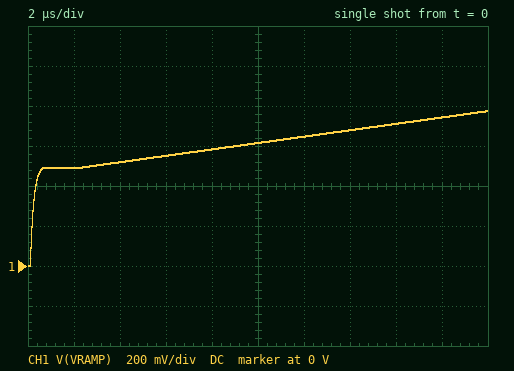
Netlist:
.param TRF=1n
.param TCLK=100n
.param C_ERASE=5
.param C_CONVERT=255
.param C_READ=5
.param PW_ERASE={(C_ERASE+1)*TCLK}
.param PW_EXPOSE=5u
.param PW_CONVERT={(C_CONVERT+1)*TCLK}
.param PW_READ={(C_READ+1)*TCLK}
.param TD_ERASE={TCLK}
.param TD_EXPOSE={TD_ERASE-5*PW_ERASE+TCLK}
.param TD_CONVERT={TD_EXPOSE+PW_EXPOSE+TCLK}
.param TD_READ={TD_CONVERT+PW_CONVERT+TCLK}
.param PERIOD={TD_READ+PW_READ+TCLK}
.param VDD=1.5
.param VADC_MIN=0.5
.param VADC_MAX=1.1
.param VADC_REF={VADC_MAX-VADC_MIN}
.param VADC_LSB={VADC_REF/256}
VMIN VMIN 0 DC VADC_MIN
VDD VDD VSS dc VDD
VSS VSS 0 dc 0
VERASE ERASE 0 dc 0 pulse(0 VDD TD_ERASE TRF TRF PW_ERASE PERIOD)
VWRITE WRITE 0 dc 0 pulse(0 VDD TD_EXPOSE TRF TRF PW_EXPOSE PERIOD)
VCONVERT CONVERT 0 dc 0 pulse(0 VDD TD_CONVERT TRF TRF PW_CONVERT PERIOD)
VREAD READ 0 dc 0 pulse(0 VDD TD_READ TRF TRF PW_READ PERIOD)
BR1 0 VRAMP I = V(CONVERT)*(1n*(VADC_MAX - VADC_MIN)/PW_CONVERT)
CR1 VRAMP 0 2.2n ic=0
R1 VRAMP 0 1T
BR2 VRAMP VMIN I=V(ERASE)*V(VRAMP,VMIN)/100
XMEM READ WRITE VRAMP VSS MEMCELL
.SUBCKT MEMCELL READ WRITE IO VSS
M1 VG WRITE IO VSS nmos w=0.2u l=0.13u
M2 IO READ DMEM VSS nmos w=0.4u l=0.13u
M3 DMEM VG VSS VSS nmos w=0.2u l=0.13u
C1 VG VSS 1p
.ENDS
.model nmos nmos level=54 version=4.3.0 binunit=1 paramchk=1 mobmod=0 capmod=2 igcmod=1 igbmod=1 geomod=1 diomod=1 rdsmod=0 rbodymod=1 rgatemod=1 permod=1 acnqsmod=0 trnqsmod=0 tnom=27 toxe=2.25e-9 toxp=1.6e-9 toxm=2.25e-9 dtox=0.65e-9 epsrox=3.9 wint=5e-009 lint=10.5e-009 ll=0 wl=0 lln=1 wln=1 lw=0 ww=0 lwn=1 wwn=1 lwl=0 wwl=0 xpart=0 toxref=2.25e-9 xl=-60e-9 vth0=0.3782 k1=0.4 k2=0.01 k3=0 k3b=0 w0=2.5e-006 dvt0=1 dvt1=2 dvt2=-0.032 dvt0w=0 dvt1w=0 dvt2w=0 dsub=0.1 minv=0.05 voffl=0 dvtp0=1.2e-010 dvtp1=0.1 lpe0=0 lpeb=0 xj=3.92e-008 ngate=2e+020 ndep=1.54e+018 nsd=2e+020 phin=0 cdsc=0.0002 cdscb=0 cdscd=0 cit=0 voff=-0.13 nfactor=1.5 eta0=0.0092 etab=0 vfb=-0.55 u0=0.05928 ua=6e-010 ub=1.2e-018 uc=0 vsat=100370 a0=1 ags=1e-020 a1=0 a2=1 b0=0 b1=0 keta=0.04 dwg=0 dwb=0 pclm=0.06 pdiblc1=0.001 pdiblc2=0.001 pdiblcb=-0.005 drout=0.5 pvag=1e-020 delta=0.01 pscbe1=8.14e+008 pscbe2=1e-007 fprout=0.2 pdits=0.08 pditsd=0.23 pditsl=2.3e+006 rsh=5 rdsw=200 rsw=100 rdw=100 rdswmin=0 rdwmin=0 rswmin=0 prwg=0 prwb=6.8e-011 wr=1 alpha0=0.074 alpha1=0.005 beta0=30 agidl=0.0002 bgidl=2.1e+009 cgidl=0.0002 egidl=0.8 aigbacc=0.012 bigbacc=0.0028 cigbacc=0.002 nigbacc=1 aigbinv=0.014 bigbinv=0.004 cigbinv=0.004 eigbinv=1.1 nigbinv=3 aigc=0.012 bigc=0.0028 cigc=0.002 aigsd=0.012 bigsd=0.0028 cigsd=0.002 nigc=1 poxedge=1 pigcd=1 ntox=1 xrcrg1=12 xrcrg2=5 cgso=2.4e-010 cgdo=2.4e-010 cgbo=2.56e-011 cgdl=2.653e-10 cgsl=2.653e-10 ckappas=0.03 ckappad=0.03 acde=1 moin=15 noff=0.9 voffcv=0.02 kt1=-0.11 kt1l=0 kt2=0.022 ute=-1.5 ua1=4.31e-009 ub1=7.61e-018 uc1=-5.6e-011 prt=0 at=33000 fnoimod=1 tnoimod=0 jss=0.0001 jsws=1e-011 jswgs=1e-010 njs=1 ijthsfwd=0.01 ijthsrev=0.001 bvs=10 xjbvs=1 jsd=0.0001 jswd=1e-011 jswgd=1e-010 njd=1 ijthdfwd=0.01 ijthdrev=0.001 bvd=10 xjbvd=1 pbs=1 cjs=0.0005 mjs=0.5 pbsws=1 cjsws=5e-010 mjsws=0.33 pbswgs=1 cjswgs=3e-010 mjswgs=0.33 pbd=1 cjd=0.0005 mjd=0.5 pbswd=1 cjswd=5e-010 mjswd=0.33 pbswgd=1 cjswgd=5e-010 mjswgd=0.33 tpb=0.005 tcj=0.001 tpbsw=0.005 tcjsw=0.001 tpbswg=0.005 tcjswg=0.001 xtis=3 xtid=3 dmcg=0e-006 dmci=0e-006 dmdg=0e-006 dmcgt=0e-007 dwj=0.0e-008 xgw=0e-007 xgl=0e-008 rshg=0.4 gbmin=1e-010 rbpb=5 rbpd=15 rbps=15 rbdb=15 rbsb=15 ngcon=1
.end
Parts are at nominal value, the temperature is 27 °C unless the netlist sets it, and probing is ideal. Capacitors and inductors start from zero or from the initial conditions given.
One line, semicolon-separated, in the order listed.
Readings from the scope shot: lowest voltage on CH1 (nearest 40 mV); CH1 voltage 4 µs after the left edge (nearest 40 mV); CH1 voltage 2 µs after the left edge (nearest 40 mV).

0 V; 520 mV; 480 mV
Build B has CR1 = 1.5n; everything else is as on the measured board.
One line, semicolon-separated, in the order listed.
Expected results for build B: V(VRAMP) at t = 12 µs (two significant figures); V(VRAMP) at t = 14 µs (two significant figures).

730 mV; 770 mV
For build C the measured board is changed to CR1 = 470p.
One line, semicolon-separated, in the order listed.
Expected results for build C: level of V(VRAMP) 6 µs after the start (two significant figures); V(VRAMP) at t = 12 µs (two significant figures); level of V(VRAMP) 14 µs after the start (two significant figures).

780 mV; 1.2 V; 1.4 V
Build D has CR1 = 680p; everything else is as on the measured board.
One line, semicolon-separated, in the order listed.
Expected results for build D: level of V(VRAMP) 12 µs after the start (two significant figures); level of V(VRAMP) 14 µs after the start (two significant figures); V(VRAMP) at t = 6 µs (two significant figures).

1.0 V; 1.1 V; 690 mV
